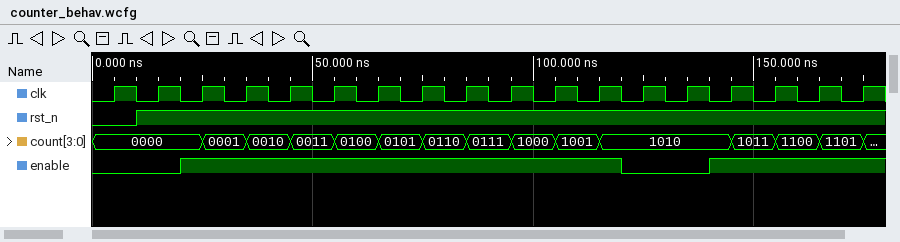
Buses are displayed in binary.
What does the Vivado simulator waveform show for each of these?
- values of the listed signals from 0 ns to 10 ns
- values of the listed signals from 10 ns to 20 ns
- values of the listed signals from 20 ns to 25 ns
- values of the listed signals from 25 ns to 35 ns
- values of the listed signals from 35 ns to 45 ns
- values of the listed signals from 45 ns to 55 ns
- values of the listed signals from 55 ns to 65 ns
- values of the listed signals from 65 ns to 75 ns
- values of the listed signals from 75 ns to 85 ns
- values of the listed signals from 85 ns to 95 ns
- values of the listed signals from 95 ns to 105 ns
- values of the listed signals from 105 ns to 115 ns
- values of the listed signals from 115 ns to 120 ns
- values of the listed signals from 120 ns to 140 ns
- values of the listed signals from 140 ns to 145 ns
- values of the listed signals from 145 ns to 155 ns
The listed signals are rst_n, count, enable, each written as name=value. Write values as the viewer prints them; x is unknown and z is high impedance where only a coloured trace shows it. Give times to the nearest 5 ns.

rst_n=0, count=0000, enable=0
rst_n=1, count=0000, enable=0
rst_n=1, count=0000, enable=1
rst_n=1, count=0001, enable=1
rst_n=1, count=0010, enable=1
rst_n=1, count=0011, enable=1
rst_n=1, count=0100, enable=1
rst_n=1, count=0101, enable=1
rst_n=1, count=0110, enable=1
rst_n=1, count=0111, enable=1
rst_n=1, count=1000, enable=1
rst_n=1, count=1001, enable=1
rst_n=1, count=1010, enable=1
rst_n=1, count=1010, enable=0
rst_n=1, count=1010, enable=1
rst_n=1, count=1011, enable=1
